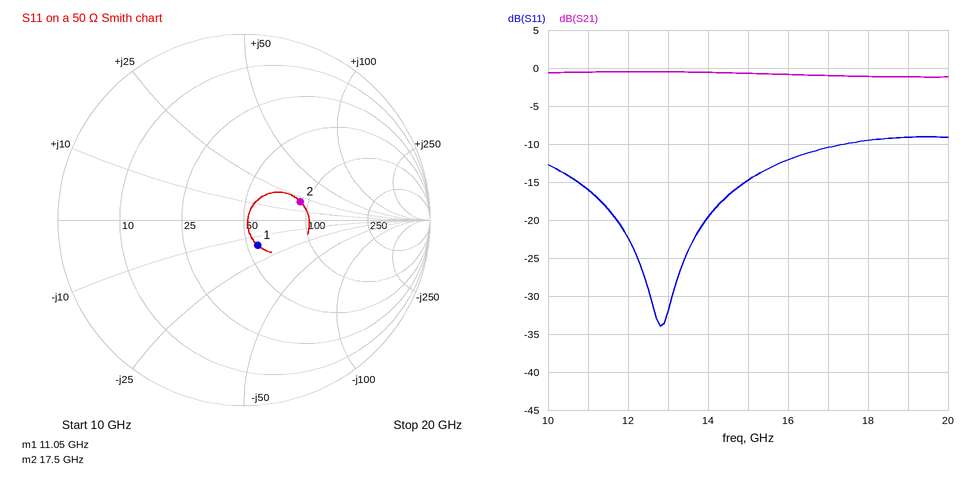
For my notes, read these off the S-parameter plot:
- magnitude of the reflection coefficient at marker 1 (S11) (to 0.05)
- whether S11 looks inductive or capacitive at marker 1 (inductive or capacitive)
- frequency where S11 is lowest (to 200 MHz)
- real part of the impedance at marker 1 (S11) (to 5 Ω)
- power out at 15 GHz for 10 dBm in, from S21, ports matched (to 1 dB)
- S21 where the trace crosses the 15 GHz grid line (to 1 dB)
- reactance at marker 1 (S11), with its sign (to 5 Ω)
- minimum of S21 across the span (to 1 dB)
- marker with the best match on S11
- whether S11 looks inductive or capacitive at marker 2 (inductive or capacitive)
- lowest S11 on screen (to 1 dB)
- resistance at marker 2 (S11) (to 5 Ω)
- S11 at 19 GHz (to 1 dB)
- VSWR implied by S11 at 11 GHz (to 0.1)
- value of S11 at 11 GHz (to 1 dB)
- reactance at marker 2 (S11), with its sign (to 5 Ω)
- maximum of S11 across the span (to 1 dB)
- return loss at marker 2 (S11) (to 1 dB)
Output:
0.15
capacitive
12.8 GHz
55 Ω
9 dBm
-1 dB
-15 Ω
-1 dB
marker 1
inductive
-34 dB
90 Ω
-9 dB
1.4
-16 dB
+20 Ω
-9 dB
10 dB
